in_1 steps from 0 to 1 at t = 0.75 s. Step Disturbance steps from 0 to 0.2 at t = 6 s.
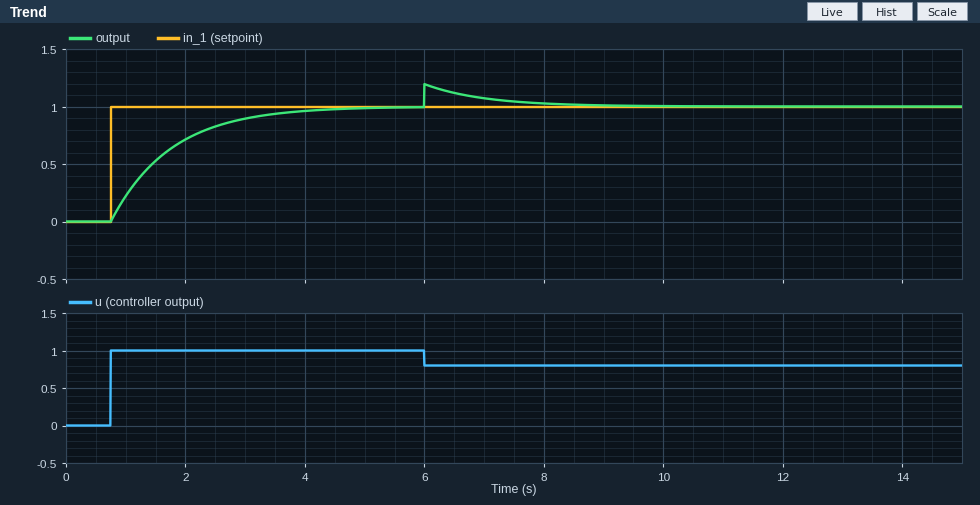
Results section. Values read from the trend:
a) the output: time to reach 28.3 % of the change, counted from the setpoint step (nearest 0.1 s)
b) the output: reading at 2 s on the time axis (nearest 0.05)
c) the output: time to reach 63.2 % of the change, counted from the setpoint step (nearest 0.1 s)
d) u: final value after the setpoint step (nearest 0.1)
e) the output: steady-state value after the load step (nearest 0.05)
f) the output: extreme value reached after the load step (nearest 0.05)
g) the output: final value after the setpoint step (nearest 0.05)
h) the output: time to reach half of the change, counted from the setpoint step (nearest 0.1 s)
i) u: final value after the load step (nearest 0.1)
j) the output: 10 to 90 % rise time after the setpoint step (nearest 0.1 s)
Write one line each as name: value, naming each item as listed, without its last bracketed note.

the output: time to reach 28.3 % of the change, counted from the setpoint step: 0.3 s
the output: reading at 2 s on the time axis: 0.70
the output: time to reach 63.2 % of the change, counted from the setpoint step: 1.0 s
u: final value after the setpoint step: 1.0
the output: steady-state value after the load step: 1.00
the output: extreme value reached after the load step: 1.20
the output: final value after the setpoint step: 1.00
the output: time to reach half of the change, counted from the setpoint step: 0.7 s
u: final value after the load step: 0.8
the output: 10 to 90 % rise time after the setpoint step: 2.2 s
